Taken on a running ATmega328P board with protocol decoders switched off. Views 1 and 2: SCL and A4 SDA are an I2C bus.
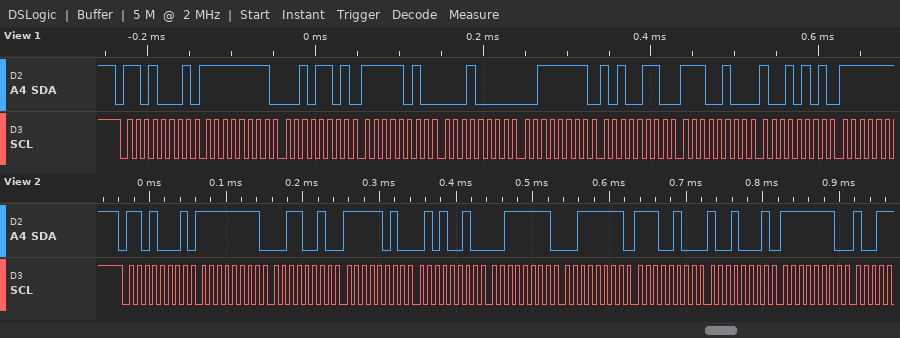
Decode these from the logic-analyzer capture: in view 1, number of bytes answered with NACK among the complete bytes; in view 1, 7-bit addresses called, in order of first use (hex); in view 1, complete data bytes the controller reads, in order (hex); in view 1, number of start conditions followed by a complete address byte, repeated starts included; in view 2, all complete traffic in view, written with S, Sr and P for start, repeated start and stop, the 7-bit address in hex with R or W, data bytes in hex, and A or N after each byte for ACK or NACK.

0
0x68
FF 2D FA 10 3F A6 E4 95
1
S 68R A FF A 32 A FA A 52 A 3F A 3F A E4 A 91 A FE A
